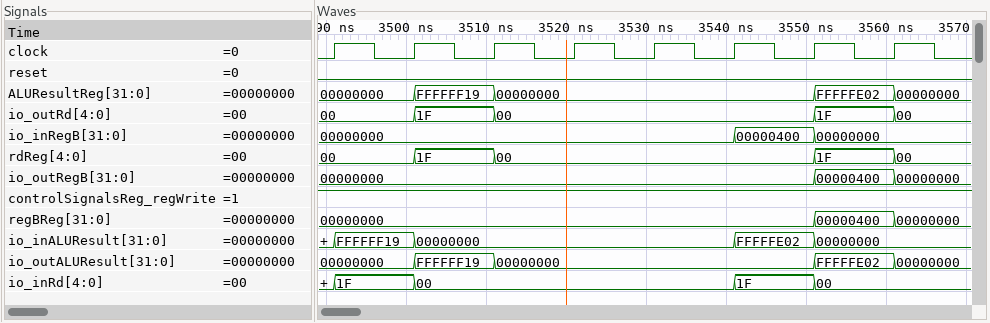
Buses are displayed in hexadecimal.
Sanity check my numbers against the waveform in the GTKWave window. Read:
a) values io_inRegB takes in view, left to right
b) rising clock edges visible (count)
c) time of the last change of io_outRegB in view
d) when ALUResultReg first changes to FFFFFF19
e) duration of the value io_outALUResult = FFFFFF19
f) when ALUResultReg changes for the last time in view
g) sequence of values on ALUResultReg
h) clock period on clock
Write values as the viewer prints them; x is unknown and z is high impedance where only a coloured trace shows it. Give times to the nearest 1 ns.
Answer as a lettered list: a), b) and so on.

a) 00000000, 00000400, 00000000
b) 8
c) 3561 ns
d) 3501 ns
e) 10 ns
f) 3561 ns
g) 00000000, FFFFFF19, 00000000, FFFFFE02, 00000000
h) 10 ns
